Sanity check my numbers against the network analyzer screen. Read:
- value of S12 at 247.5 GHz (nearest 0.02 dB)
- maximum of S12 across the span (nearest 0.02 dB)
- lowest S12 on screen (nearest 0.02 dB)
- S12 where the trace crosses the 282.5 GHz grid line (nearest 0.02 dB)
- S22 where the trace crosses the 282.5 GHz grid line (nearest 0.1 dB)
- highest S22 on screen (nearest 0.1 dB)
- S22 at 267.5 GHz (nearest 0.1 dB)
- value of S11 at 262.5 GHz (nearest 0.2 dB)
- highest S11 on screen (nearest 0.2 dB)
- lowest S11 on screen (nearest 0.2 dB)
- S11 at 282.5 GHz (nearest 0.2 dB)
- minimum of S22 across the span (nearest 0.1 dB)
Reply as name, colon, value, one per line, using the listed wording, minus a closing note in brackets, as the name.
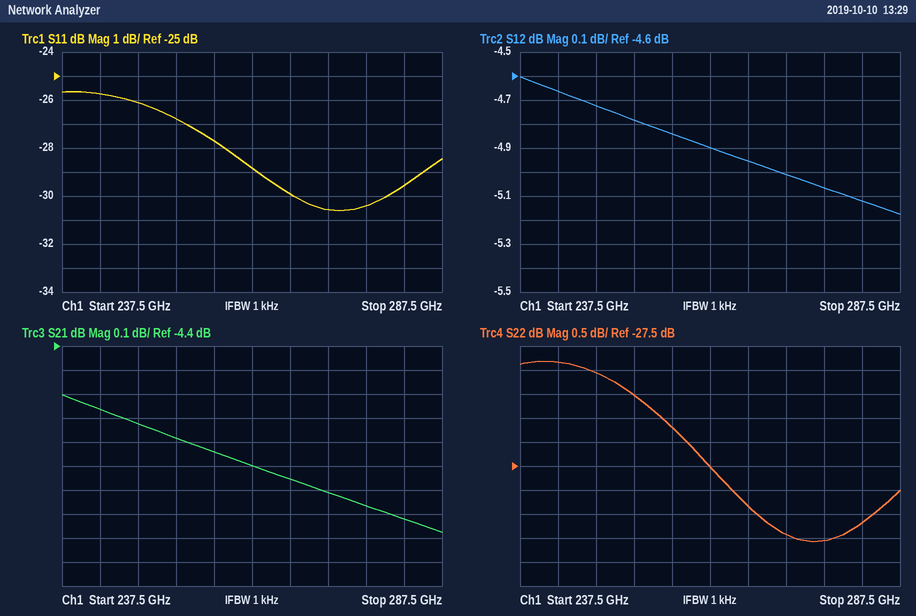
value of S12 at 247.5 GHz: -4.72 dB
maximum of S12 across the span: -4.60 dB
lowest S12 on screen: -5.18 dB
S12 where the trace crosses the 282.5 GHz grid line: -5.12 dB
S22 where the trace crosses the 282.5 GHz grid line: -28.7 dB
highest S22 on screen: -25.3 dB
S22 at 267.5 GHz: -28.3 dB
value of S11 at 262.5 GHz: -28.8 dB
highest S11 on screen: -25.6 dB
lowest S11 on screen: -30.6 dB
S11 at 282.5 GHz: -29.6 dB
minimum of S22 across the span: -29.1 dB
